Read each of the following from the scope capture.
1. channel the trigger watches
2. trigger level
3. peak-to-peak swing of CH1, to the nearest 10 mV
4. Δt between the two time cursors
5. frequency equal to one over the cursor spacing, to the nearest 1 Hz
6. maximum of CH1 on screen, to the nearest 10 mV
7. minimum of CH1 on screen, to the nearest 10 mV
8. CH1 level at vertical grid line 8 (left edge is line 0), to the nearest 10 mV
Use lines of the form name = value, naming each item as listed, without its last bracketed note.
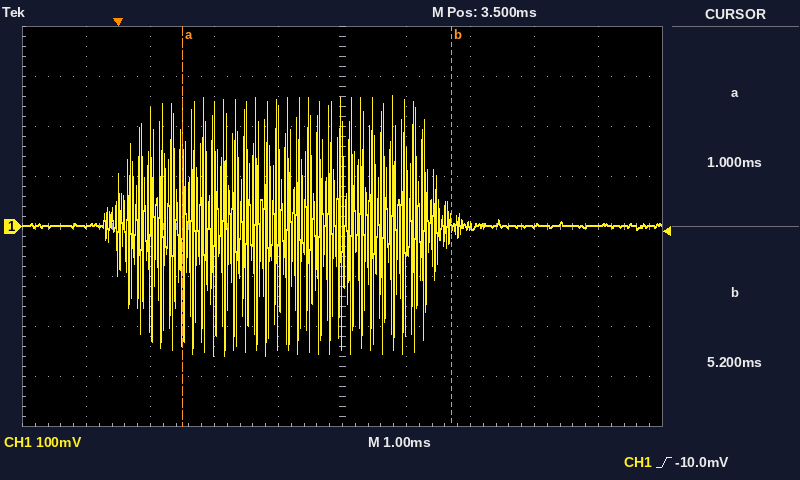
channel the trigger watches = CH1
trigger level = -10.0 mV
peak-to-peak swing of CH1, to the nearest 10 mV = 520 mV
Δt between the two time cursors = 4.2 ms
frequency equal to one over the cursor spacing, to the nearest 1 Hz = 238 Hz
maximum of CH1 on screen, to the nearest 10 mV = 260 mV
minimum of CH1 on screen, to the nearest 10 mV = -260 mV
CH1 level at vertical grid line 8 (left edge is line 0), to the nearest 10 mV = 0 mV
